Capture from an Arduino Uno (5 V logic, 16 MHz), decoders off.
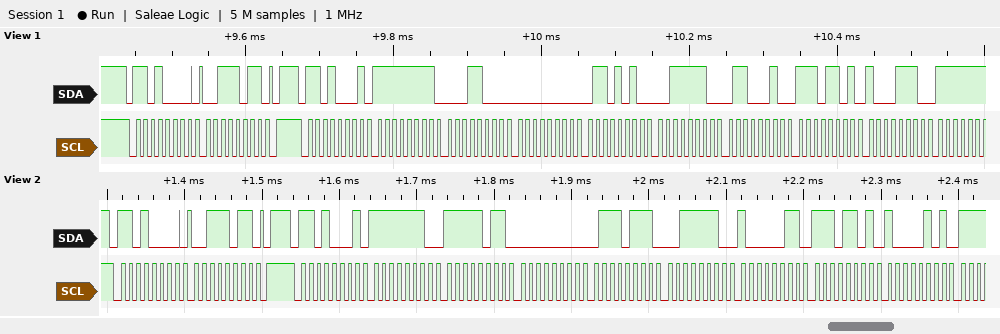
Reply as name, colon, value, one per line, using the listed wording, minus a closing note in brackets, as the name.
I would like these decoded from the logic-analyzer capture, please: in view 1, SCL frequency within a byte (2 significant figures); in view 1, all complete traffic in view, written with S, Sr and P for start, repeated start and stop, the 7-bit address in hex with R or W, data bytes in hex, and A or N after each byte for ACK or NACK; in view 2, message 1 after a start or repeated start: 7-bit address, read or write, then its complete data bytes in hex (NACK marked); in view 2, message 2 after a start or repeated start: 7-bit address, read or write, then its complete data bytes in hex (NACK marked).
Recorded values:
in view 1, SCL frequency within a byte: 100 kHz
in view 1, all complete traffic in view, written with S, Sr and P for start, repeated start and stop, the 7-bit address in hex with R or W, data bytes in hex, and A or N after each byte for ACK or NACK: S 68W A 3B A P S 68R A FF A 18 A 00 A 6A A 3E A 62 A ED A 8E A
in view 2, message 1 after a start or repeated start: 7-bit address, read or write, then its complete data bytes in hex: 0x68 write: 3B
in view 2, message 2 after a start or repeated start: 7-bit address, read or write, then its complete data bytes in hex: 0x68 read: FE FB 00 77 3E 83 ED 85
